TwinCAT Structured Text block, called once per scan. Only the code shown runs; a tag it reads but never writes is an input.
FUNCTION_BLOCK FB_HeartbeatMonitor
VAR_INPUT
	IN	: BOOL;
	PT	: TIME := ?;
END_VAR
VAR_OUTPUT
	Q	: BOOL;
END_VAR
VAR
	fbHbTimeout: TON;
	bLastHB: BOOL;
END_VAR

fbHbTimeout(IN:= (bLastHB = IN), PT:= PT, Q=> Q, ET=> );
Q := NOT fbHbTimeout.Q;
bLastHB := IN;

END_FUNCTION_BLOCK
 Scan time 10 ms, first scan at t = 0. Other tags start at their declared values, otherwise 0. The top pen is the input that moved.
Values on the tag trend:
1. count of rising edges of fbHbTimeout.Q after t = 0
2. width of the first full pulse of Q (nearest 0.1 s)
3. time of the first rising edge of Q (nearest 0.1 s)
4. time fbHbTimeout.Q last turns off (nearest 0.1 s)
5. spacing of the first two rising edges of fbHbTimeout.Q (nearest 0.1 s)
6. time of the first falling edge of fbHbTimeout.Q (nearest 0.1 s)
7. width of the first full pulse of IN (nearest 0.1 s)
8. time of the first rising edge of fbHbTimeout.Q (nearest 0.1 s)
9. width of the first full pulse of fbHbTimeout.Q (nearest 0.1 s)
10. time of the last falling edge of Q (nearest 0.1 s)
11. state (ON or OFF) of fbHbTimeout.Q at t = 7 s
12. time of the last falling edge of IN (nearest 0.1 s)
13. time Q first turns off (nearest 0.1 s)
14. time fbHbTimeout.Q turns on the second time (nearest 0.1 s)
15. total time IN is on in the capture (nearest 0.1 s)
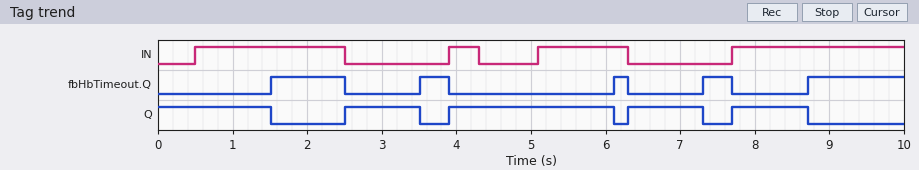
5
1.0 s
2.5 s
7.7 s
2.0 s
2.5 s
2.0 s
1.5 s
1.0 s
8.7 s
OFF
6.3 s
1.5 s
3.5 s
5.9 s
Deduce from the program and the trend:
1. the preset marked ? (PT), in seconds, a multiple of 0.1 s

1.0 s
